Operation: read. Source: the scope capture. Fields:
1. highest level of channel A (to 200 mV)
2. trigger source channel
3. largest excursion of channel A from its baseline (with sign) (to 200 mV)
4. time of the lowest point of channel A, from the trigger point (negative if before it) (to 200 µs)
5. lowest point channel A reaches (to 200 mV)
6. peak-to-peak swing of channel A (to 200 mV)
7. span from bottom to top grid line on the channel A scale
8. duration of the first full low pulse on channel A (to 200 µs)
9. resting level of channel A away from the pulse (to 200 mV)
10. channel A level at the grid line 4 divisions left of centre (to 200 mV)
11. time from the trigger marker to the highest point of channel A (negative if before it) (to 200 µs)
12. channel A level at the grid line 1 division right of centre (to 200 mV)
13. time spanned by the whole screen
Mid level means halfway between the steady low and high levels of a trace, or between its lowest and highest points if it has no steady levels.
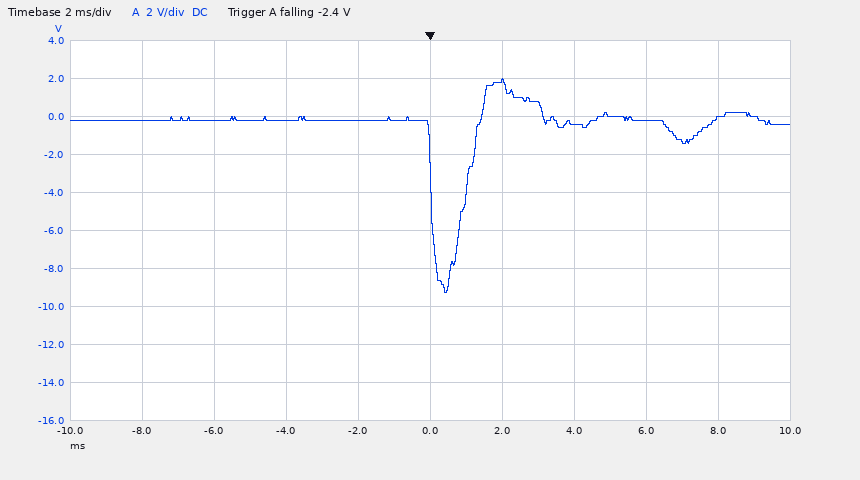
2.0 V
channel A
-9.0 V
+400 µs
-9.2 V
11.2 V
20 V
1.0 ms
-200 mV
-200 mV
+2.0 ms
1.8 V
20 ms
